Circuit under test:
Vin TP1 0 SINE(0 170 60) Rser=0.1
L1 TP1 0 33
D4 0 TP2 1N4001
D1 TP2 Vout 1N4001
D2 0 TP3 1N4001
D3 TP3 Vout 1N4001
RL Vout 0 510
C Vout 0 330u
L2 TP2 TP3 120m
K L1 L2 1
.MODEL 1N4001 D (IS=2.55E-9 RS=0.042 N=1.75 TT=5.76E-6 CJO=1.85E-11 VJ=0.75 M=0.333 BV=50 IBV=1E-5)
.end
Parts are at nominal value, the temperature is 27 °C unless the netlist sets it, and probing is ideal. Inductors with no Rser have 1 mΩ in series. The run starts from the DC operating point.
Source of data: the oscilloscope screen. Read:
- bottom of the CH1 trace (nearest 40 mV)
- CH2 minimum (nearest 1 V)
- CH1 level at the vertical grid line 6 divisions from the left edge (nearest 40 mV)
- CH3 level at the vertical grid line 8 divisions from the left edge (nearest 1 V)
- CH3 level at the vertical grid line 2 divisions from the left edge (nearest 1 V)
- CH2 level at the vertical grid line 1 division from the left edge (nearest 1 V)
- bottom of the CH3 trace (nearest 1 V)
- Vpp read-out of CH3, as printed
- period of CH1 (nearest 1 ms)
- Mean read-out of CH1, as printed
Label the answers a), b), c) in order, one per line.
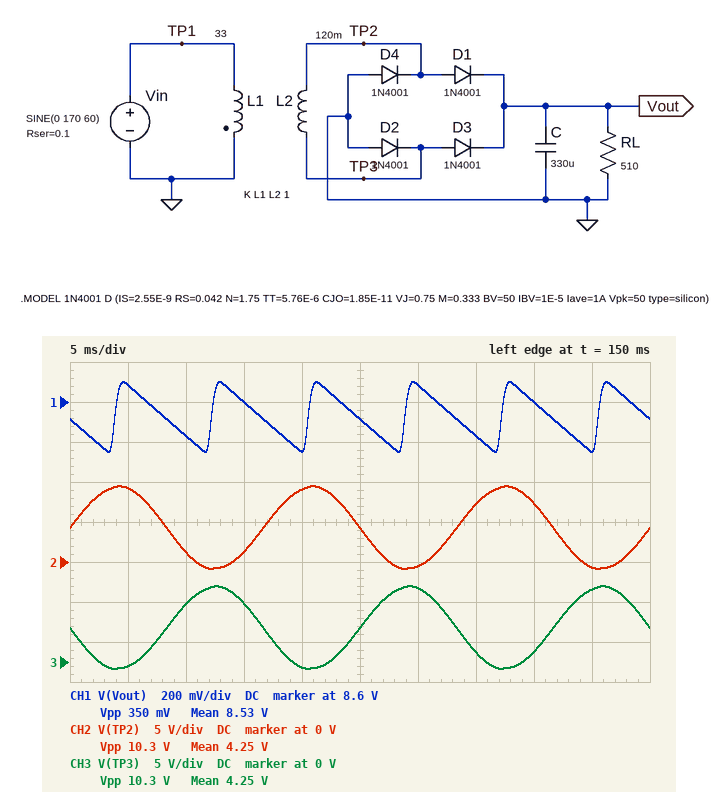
a) 8.36 V
b) -1 V
c) 8.68 V
d) 1 V
e) 7 V
f) 9 V
g) -1 V
h) 10.3 V
i) 8 ms
j) 8.53 V
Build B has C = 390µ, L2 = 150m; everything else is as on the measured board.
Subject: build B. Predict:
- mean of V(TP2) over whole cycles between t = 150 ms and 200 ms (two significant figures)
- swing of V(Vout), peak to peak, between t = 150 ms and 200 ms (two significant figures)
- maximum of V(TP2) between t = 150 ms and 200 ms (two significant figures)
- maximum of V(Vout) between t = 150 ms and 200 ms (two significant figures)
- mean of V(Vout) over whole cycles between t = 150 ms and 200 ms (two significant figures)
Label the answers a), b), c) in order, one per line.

a) 4.9 V
b) 340 mV
c) 11 V
d) 9.9 V
e) 9.7 V
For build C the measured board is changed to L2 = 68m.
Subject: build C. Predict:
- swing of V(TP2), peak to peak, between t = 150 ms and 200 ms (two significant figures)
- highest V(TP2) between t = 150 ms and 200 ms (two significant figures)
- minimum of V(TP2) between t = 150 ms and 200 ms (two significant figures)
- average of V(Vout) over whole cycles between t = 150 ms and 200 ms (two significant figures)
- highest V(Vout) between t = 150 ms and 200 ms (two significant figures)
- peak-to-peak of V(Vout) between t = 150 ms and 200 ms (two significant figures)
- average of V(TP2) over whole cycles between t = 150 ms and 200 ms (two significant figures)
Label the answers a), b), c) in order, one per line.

a) 7.7 V
b) 6.9 V
c) -810 mV
d) 6.1 V
e) 6.2 V
f) 240 mV
g) 3.0 V
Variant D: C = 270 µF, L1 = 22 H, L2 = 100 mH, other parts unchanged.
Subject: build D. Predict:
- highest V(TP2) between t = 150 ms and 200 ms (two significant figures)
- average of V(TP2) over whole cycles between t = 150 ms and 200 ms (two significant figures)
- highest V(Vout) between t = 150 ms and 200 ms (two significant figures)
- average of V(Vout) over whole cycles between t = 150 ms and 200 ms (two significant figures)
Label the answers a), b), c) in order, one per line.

a) 11 V
b) 4.8 V
c) 9.9 V
d) 9.7 V
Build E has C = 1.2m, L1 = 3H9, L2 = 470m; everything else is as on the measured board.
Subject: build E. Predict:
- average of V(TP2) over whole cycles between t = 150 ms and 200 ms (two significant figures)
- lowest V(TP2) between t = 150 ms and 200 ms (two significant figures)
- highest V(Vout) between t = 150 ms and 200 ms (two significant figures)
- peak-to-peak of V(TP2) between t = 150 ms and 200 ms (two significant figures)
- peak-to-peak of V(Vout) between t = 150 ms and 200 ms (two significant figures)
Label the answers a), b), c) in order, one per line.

a) 25 V
b) -3.8 V
c) 50 V
d) 57 V
e) 450 mV
